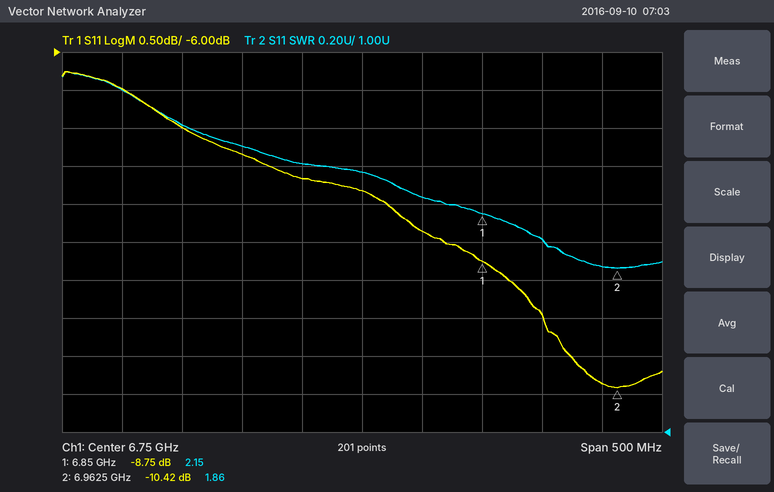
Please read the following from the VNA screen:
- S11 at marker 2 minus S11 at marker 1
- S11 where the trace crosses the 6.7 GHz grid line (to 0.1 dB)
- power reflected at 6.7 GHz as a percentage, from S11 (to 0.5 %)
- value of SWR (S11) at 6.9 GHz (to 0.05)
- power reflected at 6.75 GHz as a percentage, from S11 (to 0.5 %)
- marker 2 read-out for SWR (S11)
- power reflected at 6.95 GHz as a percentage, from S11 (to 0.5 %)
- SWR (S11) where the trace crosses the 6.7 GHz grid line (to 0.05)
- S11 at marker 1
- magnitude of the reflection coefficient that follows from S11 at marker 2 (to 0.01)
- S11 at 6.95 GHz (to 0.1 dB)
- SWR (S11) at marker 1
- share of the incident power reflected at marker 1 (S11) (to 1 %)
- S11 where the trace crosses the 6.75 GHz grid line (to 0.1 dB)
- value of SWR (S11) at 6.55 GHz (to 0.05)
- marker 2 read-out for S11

-1.67 dB
-7.7 dB
17.0 %
2.00
16.5 %
1.86
9.0 %
2.40
-8.75 dB
0.30
-10.4 dB
2.15
13 %
-7.8 dB
2.80
-10.42 dB
